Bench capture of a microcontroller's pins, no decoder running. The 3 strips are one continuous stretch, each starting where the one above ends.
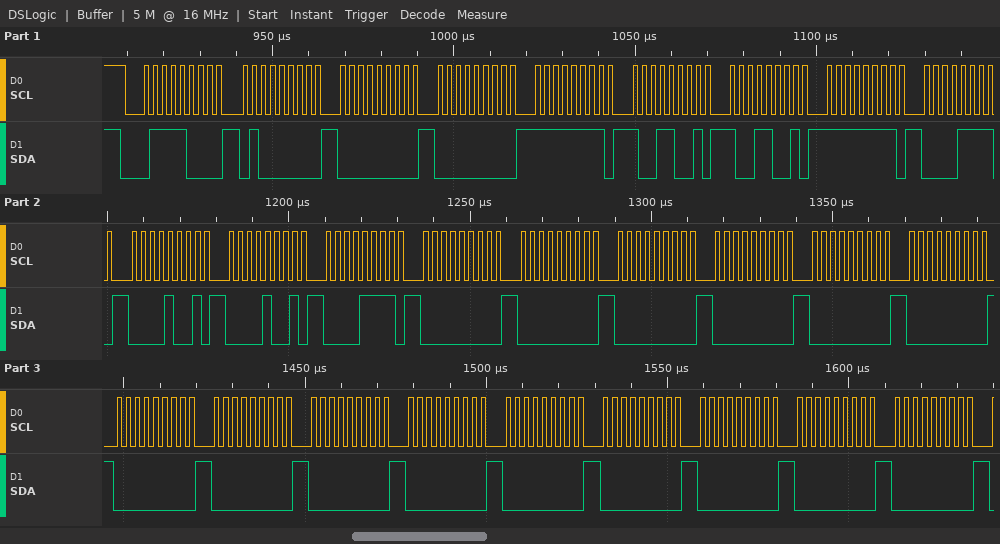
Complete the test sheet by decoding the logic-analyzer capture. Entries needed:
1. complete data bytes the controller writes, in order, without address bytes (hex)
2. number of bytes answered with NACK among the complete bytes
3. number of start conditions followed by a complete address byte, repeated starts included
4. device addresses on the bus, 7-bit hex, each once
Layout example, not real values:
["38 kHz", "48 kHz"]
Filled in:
["40 00 00 FF 99 99 FF 0F 09 09 0F 00 00 00 00 00 00 00 00 00 00 00 00 00 00 00", "0", "1", "0x3C"]
